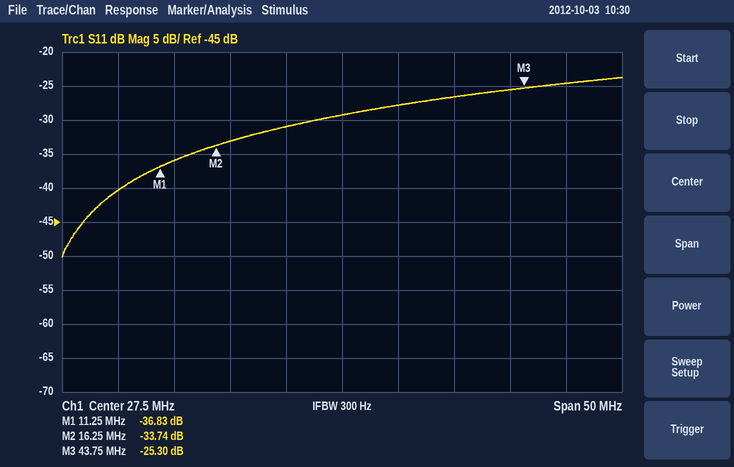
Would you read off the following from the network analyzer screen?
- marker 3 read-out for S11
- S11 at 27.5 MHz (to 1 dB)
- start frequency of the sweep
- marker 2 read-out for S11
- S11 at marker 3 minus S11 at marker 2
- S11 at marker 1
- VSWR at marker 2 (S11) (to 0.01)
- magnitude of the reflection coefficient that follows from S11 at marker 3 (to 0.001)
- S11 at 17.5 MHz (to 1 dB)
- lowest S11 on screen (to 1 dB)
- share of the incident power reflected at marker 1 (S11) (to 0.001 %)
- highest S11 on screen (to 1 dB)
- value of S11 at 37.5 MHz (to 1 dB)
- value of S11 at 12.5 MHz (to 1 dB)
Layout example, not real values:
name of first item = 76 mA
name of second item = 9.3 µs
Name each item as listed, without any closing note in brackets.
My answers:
marker 3 read-out for S11 = -25.30 dB
S11 at 27.5 MHz = -29 dB
start frequency of the sweep = 2.5 MHz
marker 2 read-out for S11 = -33.74 dB
S11 at marker 3 minus S11 at marker 2 = 8.44 dB
S11 at marker 1 = -36.83 dB
VSWR at marker 2 (S11) = 1.04
magnitude of the reflection coefficient that follows from S11 at marker 3 = 0.054
S11 at 17.5 MHz = -33 dB
lowest S11 on screen = -50 dB
share of the incident power reflected at marker 1 (S11) = 0.021 %
highest S11 on screen = -24 dB
value of S11 at 37.5 MHz = -27 dB
value of S11 at 12.5 MHz = -36 dB
